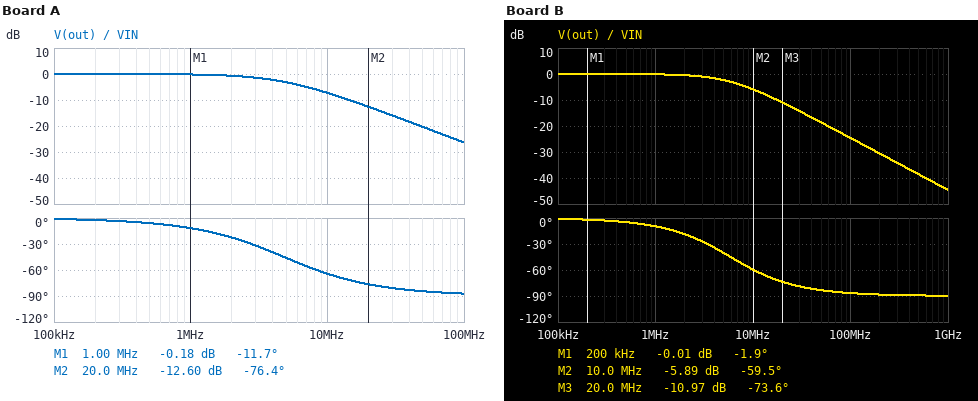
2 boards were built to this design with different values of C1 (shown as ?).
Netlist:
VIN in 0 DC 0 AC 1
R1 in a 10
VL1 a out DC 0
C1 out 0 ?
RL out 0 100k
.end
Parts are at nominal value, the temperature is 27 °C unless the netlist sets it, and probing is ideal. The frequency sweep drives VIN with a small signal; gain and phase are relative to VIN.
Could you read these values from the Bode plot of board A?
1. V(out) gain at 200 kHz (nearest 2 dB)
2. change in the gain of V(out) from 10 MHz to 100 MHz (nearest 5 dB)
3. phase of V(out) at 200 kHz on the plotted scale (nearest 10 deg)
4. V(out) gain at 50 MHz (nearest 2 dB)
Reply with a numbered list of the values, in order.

1. 0 dB
2. -20 dB
3. 0 deg
4. -20 dB
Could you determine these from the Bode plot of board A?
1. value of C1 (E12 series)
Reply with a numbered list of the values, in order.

1. 3.3 nF
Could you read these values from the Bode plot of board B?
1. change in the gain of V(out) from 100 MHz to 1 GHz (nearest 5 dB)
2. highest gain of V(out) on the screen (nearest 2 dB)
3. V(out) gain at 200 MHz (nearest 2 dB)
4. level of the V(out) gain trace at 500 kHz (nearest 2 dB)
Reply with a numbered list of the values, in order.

1. -20 dB
2. 0 dB
3. -30 dB
4. 0 dB
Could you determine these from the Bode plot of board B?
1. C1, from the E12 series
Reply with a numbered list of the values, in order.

1. 2.7 nF
